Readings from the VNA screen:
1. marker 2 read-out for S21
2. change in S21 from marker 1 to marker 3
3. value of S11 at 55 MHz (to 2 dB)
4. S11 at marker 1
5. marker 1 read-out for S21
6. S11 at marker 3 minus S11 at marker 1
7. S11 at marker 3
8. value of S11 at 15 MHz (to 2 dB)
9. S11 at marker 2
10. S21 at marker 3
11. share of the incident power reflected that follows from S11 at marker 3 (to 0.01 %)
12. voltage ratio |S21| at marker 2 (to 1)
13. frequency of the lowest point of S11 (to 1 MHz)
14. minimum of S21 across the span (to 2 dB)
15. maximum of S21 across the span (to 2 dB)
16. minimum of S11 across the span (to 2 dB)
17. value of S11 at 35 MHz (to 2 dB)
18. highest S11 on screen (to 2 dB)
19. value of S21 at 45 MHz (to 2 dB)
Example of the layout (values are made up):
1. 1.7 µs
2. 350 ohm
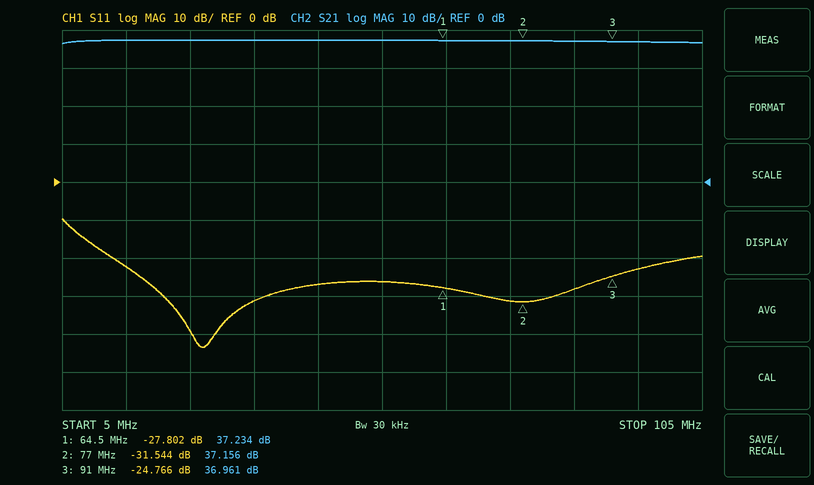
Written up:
1. 37.156 dB
2. -0.273 dB
3. -26 dB
4. -27.802 dB
5. 37.234 dB
6. 3.036 dB
7. -24.766 dB
8. -22 dB
9. -31.544 dB
10. 36.961 dB
11. 0.33 %
12. 72
13. 27 MHz
14. 36 dB
15. 38 dB
16. -44 dB
17. -32 dB
18. -10 dB
19. 38 dB
